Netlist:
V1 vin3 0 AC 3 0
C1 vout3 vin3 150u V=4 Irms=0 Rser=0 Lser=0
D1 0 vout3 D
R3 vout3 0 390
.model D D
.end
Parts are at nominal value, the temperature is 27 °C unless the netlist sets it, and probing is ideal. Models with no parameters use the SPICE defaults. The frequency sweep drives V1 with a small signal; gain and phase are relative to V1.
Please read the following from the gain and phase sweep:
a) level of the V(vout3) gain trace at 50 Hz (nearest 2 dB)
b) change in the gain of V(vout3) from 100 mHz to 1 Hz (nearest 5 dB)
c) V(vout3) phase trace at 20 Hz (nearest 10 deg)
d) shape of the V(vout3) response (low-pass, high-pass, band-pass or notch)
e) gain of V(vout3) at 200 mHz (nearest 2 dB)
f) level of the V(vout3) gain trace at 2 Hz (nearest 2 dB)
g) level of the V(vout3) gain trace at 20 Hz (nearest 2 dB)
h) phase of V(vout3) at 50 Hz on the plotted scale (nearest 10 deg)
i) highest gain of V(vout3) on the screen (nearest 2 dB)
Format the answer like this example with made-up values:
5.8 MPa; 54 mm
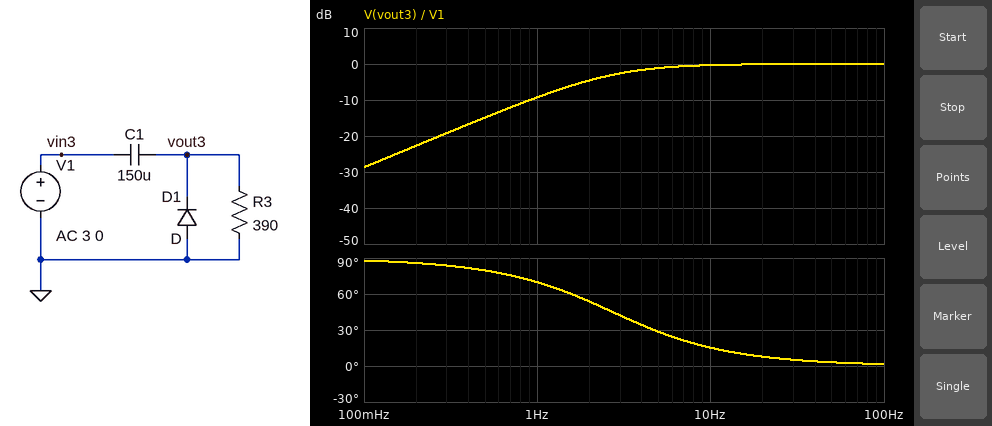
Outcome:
0 dB; 20 dB; 10 deg; high-pass; -22 dB; -4 dB; 0 dB; 0 deg; 0 dB
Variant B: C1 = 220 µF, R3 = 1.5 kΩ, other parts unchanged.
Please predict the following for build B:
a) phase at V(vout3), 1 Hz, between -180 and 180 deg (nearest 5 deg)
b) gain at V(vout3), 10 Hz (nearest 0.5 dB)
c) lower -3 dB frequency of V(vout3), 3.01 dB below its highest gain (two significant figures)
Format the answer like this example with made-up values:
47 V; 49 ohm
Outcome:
25 deg; 0 dB; 480 mHz
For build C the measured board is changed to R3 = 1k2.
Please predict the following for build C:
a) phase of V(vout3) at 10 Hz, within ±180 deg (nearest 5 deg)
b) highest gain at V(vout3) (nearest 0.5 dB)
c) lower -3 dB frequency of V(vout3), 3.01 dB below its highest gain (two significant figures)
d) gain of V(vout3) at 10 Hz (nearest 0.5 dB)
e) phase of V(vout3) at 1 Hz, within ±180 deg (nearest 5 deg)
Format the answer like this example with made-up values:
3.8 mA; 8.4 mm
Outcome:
5 deg; 0 dB; 880 mHz; 0 dB; 40 deg
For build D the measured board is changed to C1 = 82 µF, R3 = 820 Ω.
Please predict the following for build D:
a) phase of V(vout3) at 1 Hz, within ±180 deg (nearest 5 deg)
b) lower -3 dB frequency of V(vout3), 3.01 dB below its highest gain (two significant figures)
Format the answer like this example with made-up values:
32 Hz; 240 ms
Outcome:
65 deg; 2.4 Hz
